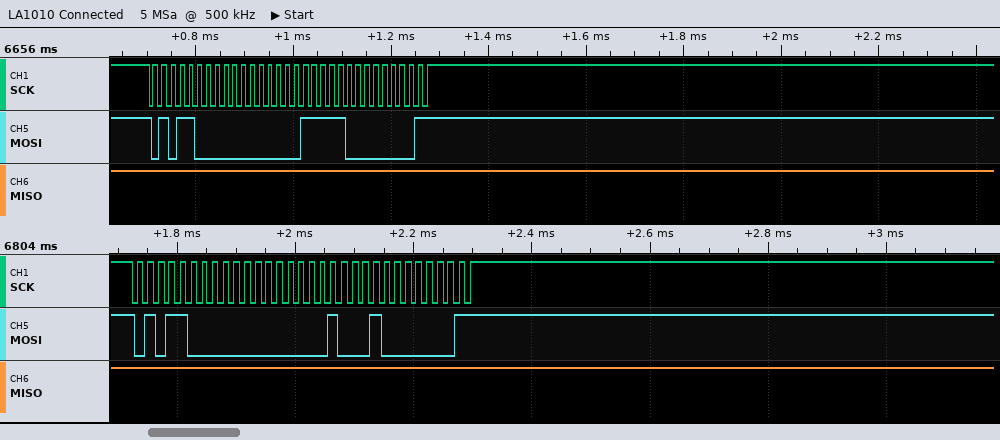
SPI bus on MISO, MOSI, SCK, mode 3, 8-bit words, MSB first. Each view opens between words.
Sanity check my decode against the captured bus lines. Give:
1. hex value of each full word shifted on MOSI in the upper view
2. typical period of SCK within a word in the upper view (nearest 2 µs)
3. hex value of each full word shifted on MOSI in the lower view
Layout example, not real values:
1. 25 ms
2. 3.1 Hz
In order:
1. 58, 00, 7C, 03
2. 18 µs
3. 58, 00, 22, 03
